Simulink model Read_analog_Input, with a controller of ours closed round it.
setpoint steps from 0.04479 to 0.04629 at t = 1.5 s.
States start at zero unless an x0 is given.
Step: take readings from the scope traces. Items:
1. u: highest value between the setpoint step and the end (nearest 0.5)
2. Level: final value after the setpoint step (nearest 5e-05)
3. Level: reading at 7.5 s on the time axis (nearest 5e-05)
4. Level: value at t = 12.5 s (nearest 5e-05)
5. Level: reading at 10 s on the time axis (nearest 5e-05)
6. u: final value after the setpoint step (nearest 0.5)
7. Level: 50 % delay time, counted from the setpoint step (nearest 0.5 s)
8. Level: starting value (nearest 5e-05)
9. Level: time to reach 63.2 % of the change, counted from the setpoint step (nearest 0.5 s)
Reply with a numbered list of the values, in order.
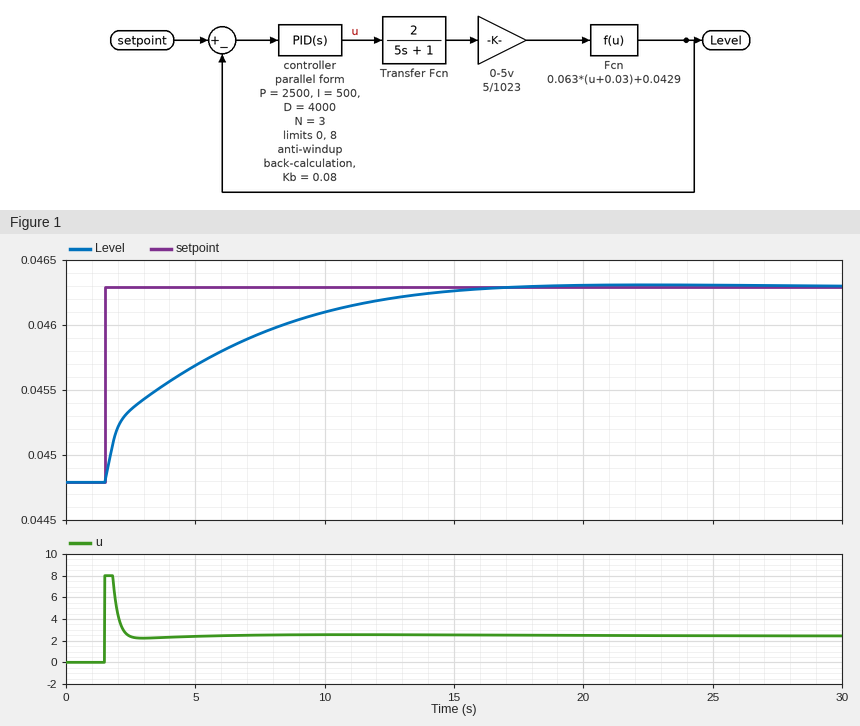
1. 8.0
2. 0.04630
3. 0.04595
4. 0.04620
5. 0.04610
6. 2.5
7. 2.5 s
8. 0.04480
9. 4.0 s
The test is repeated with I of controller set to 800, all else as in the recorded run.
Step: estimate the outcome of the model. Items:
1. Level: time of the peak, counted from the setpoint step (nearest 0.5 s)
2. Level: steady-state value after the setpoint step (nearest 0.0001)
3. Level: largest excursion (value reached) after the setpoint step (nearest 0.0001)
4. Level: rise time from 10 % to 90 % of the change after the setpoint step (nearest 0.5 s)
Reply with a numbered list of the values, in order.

1. 13.0 s
2. 0.0463
3. 0.0464
4. 6.5 s
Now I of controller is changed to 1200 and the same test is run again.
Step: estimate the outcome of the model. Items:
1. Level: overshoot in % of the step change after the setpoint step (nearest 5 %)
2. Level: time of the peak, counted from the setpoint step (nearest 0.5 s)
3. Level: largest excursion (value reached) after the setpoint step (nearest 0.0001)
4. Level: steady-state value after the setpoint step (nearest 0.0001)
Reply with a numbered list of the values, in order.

1. 10 %
2. 10.0 s
3. 0.0465
4. 0.0463
